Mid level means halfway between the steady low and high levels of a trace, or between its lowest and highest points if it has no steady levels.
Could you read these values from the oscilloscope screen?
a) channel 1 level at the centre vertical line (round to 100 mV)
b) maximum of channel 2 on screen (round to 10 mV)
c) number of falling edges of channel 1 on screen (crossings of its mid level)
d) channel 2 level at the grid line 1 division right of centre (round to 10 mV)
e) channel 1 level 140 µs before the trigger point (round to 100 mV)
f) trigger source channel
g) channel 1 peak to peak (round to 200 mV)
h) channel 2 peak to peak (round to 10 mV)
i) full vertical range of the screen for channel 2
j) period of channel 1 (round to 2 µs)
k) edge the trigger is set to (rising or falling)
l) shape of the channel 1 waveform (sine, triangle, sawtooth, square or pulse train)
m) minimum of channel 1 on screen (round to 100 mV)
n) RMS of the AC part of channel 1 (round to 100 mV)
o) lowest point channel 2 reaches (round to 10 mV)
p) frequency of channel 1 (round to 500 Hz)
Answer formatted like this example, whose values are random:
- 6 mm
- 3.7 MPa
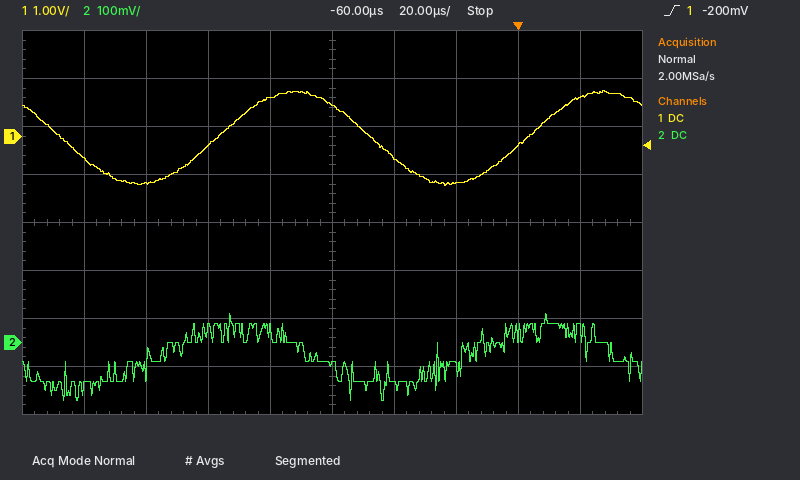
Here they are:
- 700 mV
- 60 mV
- 2
- -90 mV
- -500 mV
- channel 1
- 2.0 V
- 180 mV
- 800 mV
- 100 µs
- rising
- sine
- -1.0 V
- 700 mV
- -120 mV
- 10.0 kHz
